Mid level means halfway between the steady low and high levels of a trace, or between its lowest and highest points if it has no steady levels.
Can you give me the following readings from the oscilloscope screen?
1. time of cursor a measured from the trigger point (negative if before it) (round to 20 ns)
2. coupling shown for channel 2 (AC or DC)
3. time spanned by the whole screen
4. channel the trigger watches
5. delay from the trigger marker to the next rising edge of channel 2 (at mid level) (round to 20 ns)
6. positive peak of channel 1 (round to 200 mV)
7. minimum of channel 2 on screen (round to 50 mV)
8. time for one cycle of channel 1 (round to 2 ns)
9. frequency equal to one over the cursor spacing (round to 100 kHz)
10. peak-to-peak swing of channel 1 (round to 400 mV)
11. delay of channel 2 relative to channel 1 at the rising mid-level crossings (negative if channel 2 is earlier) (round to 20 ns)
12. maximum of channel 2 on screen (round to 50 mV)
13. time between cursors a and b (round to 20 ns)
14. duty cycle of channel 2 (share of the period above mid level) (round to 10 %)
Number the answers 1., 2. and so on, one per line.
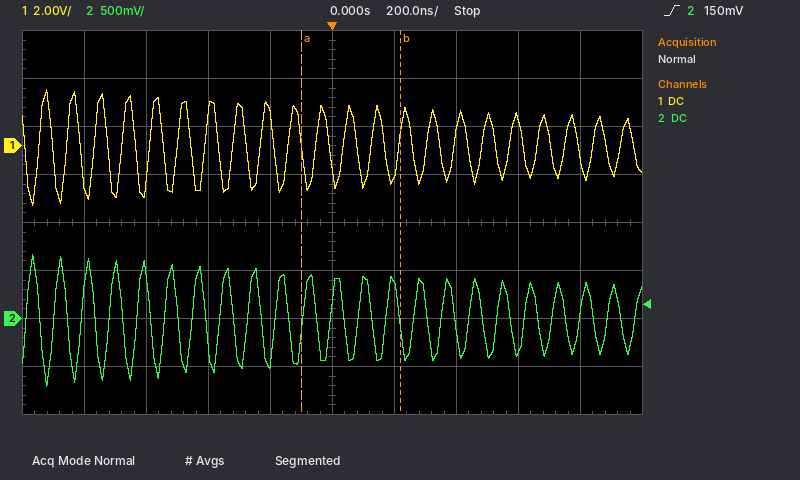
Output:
1. -100 ns
2. DC
3. 2 µs
4. channel 2
5. 80 ns
6. 2.4 V
7. -700 mV
8. 90 ns
9. 3.1 MHz
10. 4.8 V
11. -40 ns
12. 650 mV
13. 320 ns
14. 50 %
